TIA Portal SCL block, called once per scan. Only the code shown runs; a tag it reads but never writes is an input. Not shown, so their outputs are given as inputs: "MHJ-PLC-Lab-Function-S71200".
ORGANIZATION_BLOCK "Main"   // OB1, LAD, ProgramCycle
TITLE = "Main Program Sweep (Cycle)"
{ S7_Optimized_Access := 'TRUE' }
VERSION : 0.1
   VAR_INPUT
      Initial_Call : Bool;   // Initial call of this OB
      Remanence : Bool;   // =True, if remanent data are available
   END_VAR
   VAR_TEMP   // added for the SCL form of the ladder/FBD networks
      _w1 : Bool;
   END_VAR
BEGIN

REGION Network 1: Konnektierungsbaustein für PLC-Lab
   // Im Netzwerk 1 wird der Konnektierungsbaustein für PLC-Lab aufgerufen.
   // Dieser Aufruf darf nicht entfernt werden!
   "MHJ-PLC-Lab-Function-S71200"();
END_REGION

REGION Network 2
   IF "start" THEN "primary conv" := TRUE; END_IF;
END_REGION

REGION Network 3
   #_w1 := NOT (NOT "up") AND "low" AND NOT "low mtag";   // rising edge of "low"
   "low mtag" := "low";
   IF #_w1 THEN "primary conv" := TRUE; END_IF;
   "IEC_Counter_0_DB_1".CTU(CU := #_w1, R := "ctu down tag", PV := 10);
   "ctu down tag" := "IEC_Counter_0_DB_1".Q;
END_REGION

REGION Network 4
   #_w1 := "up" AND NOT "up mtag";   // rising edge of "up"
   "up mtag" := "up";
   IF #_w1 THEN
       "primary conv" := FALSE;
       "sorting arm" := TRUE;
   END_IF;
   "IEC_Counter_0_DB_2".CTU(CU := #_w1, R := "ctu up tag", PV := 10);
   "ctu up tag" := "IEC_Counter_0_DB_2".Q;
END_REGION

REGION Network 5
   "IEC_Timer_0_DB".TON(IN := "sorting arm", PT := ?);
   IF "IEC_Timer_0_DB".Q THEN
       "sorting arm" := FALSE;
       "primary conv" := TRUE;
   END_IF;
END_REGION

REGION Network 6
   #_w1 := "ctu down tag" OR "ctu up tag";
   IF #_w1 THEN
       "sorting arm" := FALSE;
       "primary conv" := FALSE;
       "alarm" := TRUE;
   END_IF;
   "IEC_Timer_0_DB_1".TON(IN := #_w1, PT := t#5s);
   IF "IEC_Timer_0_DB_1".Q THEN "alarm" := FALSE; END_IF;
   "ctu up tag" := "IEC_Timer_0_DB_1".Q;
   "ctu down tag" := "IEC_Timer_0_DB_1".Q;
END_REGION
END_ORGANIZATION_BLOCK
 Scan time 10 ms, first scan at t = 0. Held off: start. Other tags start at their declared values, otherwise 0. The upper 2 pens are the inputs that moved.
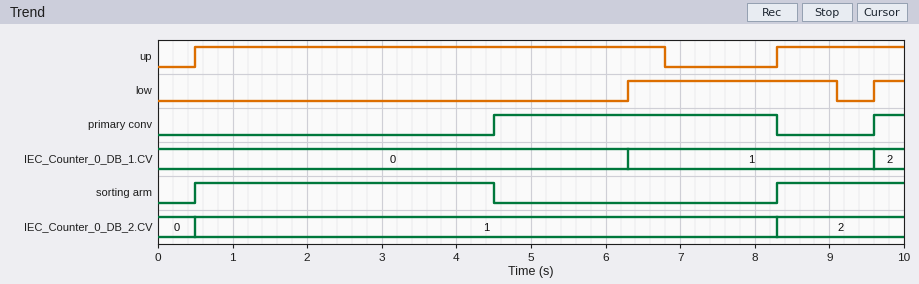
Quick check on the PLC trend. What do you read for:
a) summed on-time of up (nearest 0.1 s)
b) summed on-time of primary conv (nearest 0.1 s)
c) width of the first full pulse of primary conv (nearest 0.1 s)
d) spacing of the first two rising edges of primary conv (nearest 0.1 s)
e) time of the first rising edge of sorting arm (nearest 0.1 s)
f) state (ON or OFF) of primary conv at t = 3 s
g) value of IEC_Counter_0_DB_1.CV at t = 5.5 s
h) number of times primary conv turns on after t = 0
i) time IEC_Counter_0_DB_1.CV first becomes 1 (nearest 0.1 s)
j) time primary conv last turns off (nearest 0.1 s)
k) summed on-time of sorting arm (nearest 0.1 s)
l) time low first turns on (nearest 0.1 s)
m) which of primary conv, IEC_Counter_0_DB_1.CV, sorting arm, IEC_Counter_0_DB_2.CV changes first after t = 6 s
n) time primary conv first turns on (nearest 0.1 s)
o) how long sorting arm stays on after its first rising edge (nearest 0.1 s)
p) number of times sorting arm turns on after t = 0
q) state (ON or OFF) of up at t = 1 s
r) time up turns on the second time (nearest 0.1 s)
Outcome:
8.0 s
4.2 s
3.8 s
5.1 s
0.5 s
OFF
0
2
6.3 s
8.3 s
5.7 s
6.3 s
IEC_Counter_0_DB_1.CV
4.5 s
4.0 s
2
ON
8.3 s
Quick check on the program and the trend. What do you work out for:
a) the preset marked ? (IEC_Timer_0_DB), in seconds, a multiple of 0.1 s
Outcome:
4.0 s
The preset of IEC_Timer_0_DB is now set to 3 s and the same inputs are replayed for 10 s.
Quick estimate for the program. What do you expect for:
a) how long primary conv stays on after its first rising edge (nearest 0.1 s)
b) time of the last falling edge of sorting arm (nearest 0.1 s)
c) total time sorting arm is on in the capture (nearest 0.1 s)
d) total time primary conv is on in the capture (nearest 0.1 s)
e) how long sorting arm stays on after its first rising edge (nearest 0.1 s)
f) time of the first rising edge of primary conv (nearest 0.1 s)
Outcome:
4.8 s
3.5 s
4.7 s
5.2 s
3.0 s
3.5 s
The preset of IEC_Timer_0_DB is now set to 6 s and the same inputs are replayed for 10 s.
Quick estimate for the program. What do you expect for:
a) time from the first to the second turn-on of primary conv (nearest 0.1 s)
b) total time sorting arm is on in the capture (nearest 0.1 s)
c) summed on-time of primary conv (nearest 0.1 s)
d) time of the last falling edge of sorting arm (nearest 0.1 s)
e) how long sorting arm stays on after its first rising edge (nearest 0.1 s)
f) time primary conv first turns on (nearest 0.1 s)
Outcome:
3.3 s
7.7 s
2.4 s
6.5 s
6.0 s
6.3 s
